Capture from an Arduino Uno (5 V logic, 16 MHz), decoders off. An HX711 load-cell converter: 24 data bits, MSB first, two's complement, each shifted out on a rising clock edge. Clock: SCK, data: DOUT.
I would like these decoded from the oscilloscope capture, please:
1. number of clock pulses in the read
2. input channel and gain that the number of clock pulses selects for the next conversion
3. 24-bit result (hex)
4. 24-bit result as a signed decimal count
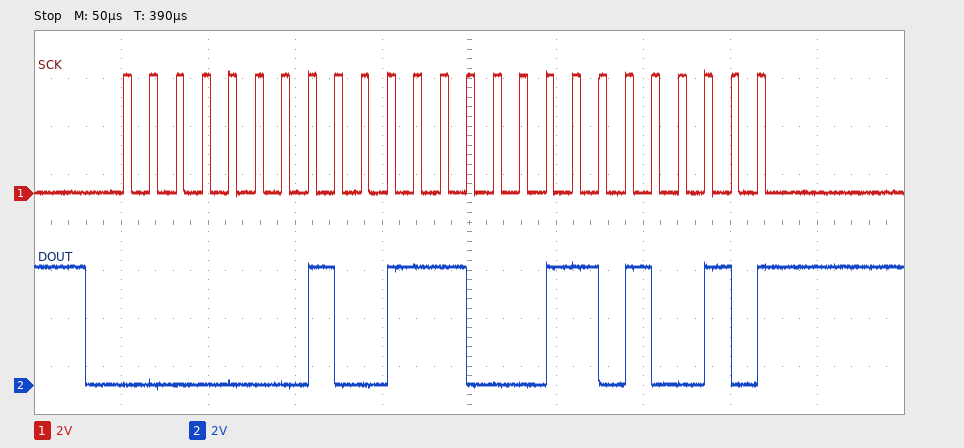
25
channel A, gain 128
0x0138D2
80082
